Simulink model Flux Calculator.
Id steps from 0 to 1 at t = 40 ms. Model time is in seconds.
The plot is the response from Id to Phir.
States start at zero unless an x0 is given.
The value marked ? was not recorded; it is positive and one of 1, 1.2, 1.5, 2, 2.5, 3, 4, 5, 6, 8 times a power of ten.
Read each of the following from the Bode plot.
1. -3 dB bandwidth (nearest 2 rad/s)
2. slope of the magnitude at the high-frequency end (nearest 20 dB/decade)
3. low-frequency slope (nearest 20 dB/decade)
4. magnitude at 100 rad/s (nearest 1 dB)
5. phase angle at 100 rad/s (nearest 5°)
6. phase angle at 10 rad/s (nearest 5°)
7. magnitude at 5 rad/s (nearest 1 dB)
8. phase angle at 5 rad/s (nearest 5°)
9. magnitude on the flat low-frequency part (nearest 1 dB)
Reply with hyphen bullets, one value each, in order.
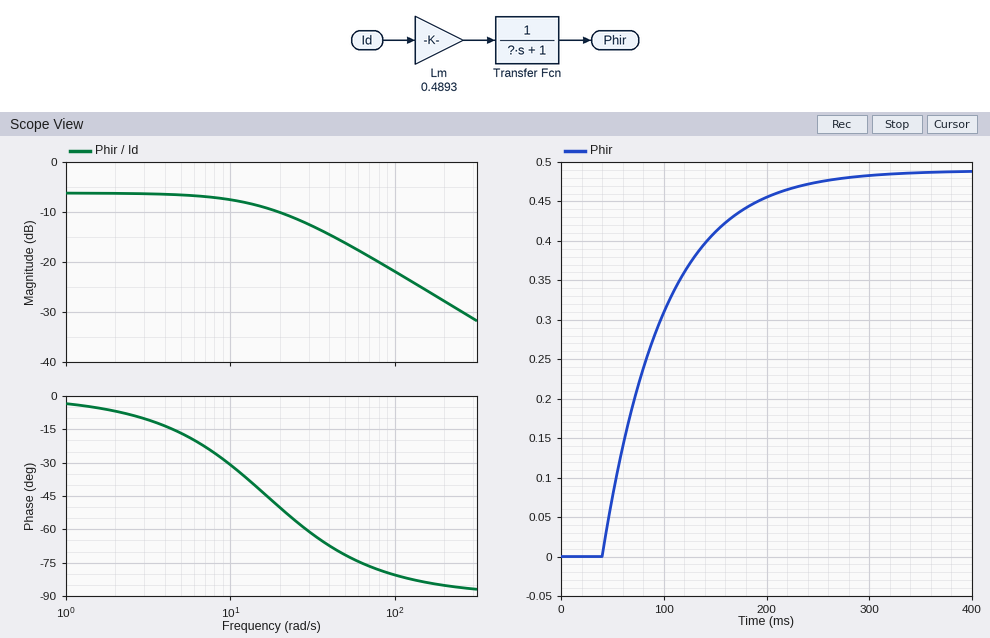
- 16 rad/s
- -20 dB/decade
- 0 dB/decade
- -22 dB
- -80°
- -30°
- -7 dB
- -15°
- -6 dB
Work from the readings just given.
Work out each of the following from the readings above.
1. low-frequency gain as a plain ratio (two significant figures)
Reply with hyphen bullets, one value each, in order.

- 0.50
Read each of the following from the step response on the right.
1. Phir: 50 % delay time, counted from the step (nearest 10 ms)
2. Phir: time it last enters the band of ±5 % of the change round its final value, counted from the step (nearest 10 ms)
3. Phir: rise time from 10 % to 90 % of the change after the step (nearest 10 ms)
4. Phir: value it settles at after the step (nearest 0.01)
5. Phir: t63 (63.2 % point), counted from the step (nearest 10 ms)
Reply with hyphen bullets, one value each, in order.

- 40 ms
- 180 ms
- 130 ms
- 0.49
- 60 ms
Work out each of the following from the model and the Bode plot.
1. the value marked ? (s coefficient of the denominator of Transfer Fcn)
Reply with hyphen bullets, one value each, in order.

- 0.06
